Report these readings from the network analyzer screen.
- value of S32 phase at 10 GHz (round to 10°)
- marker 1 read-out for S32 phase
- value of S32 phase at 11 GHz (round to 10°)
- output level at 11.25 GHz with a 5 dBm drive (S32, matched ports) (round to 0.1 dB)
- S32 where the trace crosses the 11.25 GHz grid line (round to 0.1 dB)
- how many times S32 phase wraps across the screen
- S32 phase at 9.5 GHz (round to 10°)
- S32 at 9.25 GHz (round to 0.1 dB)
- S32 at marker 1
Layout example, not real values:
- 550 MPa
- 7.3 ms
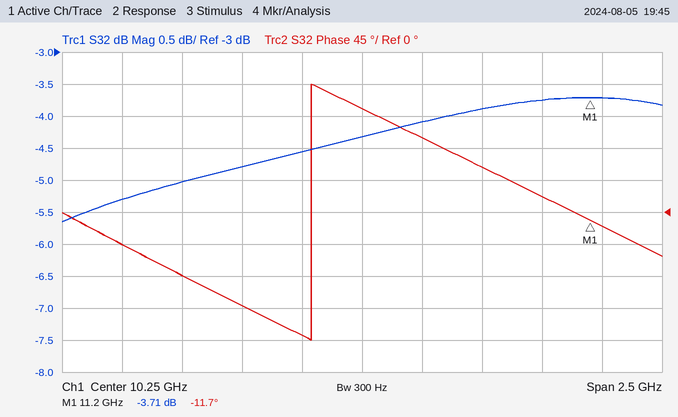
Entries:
- -170°
- -11.7°
- 20°
- 1.3 dBm
- -3.7 dB
- 1
- -90°
- -5.3 dB
- -3.71 dB
